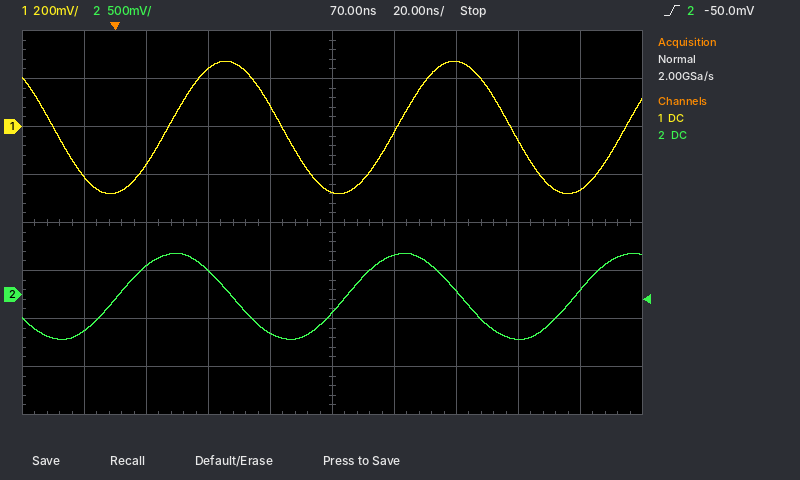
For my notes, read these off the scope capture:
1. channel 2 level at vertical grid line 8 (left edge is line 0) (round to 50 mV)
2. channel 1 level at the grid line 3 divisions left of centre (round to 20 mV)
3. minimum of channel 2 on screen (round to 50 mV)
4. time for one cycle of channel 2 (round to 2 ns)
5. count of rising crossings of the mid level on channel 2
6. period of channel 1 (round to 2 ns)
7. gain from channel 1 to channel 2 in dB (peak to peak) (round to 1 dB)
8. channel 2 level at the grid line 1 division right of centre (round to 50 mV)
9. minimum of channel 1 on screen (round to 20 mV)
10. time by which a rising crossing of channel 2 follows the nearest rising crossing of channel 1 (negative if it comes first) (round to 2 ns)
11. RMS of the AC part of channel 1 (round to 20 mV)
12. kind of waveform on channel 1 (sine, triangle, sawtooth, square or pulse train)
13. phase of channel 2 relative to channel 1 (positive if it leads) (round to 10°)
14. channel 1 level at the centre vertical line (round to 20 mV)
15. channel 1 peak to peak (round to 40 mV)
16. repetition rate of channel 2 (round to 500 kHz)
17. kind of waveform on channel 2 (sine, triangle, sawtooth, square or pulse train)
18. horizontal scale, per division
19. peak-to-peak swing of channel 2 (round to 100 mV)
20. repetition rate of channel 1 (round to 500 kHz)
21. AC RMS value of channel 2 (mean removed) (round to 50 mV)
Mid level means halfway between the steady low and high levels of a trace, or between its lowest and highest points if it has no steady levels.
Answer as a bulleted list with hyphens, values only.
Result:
- -450 mV
- -160 mV
- -450 mV
- 74 ns
- 3
- 74 ns
- 4 dB
- 400 mV
- -280 mV
- -16 ns
- 200 mV
- sine
- +80°
- -280 mV
- 560 mV
- 13.5 MHz
- sine
- 20 ns
- 900 mV
- 13.5 MHz
- 300 mV
